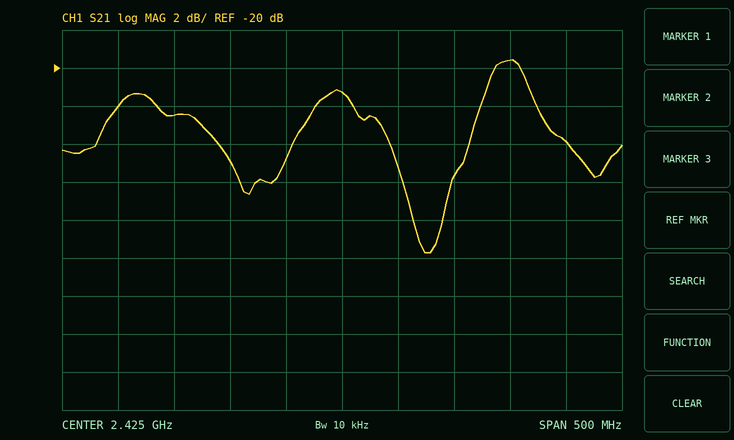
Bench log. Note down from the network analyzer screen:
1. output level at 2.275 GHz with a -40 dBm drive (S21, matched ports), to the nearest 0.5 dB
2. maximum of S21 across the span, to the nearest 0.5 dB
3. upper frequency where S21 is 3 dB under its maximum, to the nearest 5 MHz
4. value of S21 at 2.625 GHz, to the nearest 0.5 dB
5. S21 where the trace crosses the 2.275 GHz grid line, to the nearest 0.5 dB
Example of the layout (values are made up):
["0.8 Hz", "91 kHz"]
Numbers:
["-62.5 dBm", "-19.5 dB", "2.605 GHz", "-24.0 dB", "-22.5 dB"]
